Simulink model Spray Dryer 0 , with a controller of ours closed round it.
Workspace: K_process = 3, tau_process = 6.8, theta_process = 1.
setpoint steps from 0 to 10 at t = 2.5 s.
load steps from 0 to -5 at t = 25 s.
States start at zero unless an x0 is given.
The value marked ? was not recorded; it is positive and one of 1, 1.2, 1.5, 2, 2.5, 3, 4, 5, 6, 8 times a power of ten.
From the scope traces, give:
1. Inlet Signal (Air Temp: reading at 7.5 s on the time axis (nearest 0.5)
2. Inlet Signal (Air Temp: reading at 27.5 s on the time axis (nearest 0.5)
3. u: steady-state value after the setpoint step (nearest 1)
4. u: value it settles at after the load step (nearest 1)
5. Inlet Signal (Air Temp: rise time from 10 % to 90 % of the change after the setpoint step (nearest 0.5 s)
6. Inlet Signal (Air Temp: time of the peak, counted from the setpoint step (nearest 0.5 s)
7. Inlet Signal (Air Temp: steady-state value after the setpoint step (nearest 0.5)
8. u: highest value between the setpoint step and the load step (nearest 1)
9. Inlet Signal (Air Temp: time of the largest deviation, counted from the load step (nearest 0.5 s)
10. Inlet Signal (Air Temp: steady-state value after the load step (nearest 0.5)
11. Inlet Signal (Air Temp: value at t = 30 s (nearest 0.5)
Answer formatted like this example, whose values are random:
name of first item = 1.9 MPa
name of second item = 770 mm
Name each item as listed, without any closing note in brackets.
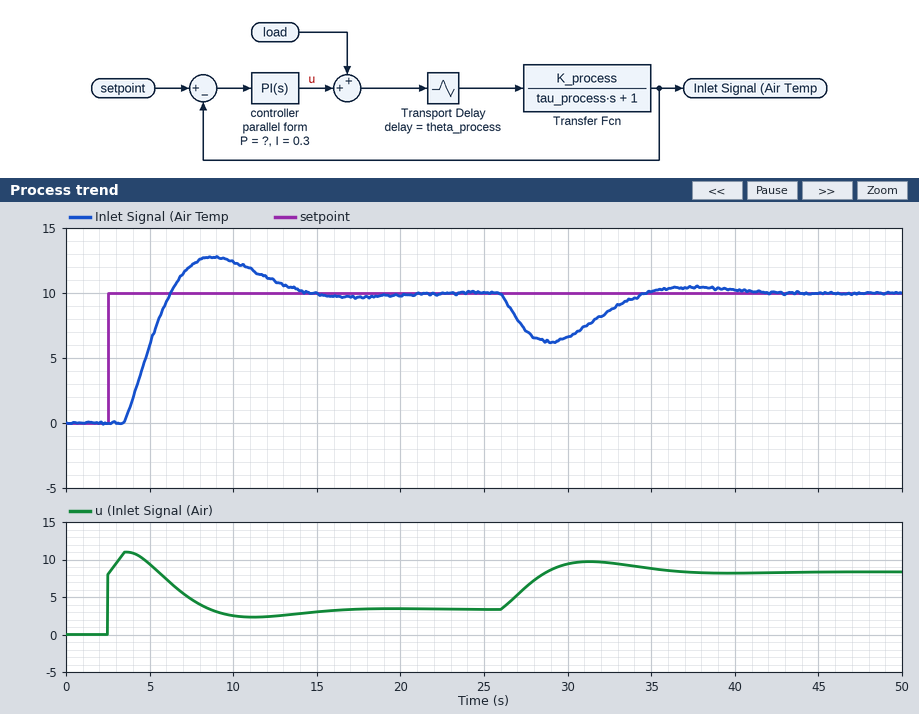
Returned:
Inlet Signal (Air Temp: reading at 7.5 s on the time axis = 12.0
Inlet Signal (Air Temp: reading at 27.5 s on the time axis = 7.0
u: steady-state value after the setpoint step = 3
u: value it settles at after the load step = 8
Inlet Signal (Air Temp: rise time from 10 % to 90 % of the change after the setpoint step = 2.0 s
Inlet Signal (Air Temp: time of the peak, counted from the setpoint step = 6.5 s
Inlet Signal (Air Temp: steady-state value after the setpoint step = 10.0
u: highest value between the setpoint step and the load step = 11
Inlet Signal (Air Temp: time of the largest deviation, counted from the load step = 4.0 s
Inlet Signal (Air Temp: steady-state value after the load step = 10.0
Inlet Signal (Air Temp: value at t = 30 s = 6.5
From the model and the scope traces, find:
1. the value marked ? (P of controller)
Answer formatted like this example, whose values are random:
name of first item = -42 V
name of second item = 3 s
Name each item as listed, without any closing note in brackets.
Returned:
the value marked ? = 0.8
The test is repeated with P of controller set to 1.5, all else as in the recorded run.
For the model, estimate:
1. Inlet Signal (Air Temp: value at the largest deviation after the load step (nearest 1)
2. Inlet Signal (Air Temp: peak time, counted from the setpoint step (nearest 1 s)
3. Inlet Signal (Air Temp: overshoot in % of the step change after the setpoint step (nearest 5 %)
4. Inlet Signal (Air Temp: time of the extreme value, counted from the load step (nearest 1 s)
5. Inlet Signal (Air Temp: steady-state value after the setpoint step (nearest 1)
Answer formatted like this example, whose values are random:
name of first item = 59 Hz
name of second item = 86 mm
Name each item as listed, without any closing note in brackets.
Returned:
Inlet Signal (Air Temp: value at the largest deviation after the load step = 7
Inlet Signal (Air Temp: peak time, counted from the setpoint step = 4 s
Inlet Signal (Air Temp: overshoot in % of the step change after the setpoint step = 25 %
Inlet Signal (Air Temp: time of the extreme value, counted from the load step = 3 s
Inlet Signal (Air Temp: steady-state value after the setpoint step = 10
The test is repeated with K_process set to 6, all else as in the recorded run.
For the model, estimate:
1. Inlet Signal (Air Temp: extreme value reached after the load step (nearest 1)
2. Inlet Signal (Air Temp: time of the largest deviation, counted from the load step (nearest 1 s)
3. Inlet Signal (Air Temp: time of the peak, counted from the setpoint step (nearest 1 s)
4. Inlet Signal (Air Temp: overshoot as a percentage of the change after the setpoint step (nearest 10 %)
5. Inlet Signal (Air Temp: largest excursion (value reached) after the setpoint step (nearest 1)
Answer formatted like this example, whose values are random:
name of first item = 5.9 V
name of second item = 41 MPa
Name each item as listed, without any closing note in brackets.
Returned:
Inlet Signal (Air Temp: extreme value reached after the load step = 4
Inlet Signal (Air Temp: time of the largest deviation, counted from the load step = 3 s
Inlet Signal (Air Temp: time of the peak, counted from the setpoint step = 4 s
Inlet Signal (Air Temp: overshoot as a percentage of the change after the setpoint step = 50 %
Inlet Signal (Air Temp: largest excursion (value reached) after the setpoint step = 15
